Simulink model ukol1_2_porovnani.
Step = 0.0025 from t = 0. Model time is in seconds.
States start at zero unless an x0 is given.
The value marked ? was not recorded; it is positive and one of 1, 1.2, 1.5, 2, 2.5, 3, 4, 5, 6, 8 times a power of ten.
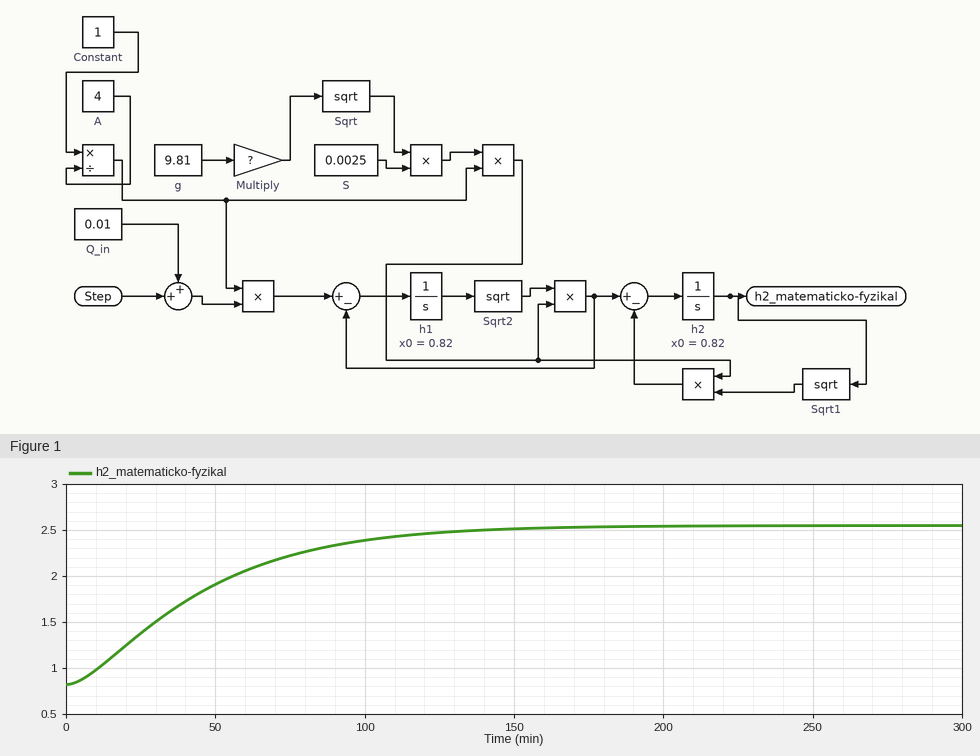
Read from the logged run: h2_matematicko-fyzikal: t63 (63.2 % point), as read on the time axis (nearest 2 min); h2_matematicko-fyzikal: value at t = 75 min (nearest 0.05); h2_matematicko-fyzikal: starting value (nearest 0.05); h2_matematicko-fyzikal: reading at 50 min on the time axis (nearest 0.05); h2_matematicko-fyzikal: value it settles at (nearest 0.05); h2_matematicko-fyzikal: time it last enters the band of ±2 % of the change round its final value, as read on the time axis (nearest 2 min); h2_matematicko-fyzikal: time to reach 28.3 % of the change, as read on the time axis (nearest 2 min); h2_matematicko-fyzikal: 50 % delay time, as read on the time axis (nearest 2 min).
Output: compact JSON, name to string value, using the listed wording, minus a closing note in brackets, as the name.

{"h2_matematicko-fyzikal: t63 (63.2 % point), as read on the time axis": "50 min", "h2_matematicko-fyzikal: value at t = 75 min": "2.20", "h2_matematicko-fyzikal: starting value": "0.80", "h2_matematicko-fyzikal: reading at 50 min on the time axis": "1.90", "h2_matematicko-fyzikal: value it settles at": "2.55", "h2_matematicko-fyzikal: time it last enters the band of ±2 % of the change round its final value, as read on the time axis": "152 min", "h2_matematicko-fyzikal: time to reach 28.3 % of the change, as read on the time axis": "22 min", "h2_matematicko-fyzikal: 50 % delay time, as read on the time axis": "38 min"}
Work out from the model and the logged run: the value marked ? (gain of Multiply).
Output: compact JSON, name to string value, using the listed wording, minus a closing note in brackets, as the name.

{"the value marked ?": "1"}
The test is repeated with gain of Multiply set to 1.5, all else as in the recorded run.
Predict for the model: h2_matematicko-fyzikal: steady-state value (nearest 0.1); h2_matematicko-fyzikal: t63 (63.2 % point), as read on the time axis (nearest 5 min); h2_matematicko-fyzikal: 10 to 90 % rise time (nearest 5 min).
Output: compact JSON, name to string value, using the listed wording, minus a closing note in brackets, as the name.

{"h2_matematicko-fyzikal: steady-state value": "1.7", "h2_matematicko-fyzikal: t63 (63.2 % point), as read on the time axis": "35 min", "h2_matematicko-fyzikal: 10 to 90 % rise time": "60 min"}
